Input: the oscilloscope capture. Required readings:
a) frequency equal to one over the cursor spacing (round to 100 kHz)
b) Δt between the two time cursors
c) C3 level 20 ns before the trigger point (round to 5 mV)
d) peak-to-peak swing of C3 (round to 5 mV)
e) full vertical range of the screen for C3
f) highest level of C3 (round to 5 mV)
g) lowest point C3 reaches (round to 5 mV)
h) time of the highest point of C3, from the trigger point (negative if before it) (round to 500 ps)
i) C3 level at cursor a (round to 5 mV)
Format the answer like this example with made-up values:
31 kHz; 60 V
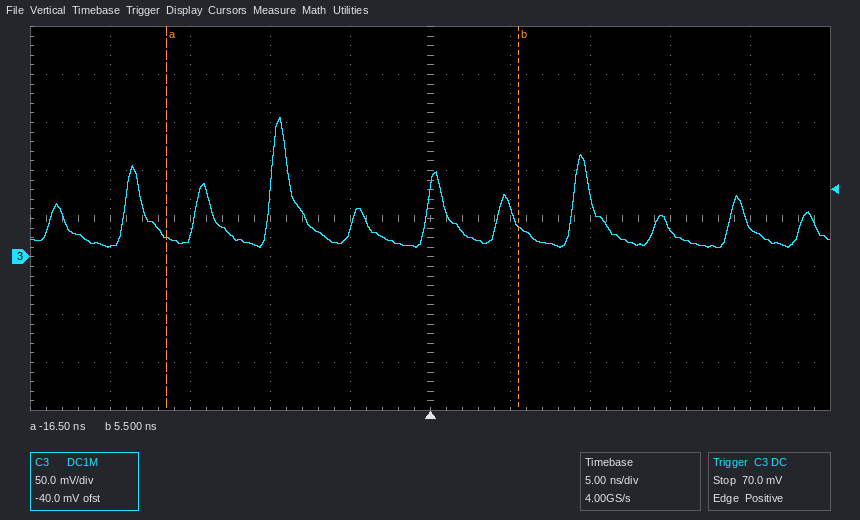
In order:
45.5 MHz; 22.0 ns; 10 mV; 135 mV; 400 mV; 145 mV; 10 mV; -9.5 ns; 20 mV
